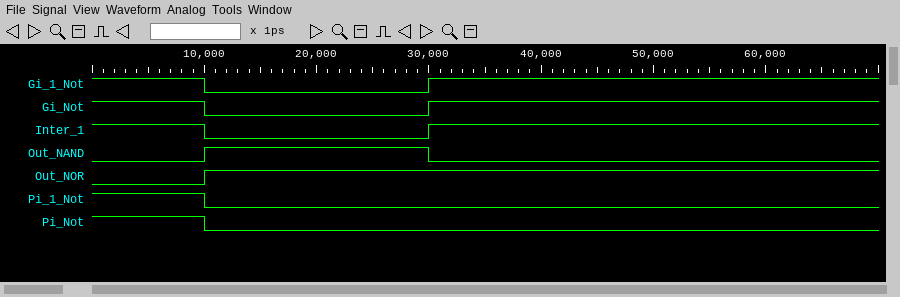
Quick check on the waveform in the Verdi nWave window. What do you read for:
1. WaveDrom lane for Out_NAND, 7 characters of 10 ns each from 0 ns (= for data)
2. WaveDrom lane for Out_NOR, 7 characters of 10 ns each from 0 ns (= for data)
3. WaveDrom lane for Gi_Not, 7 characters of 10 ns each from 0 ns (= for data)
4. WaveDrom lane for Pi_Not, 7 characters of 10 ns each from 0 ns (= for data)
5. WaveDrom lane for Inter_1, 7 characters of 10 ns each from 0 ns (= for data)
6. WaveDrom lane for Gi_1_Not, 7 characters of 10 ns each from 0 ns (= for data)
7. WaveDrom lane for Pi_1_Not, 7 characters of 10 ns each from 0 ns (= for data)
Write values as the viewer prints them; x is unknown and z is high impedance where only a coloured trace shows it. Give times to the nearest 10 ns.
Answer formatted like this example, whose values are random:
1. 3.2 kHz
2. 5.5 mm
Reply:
1. {name: 'Out_NAND', wave: '01.0...'}
2. {name: 'Out_NOR', wave: '01.....'}
3. {name: 'Gi_Not', wave: '10.1...'}
4. {name: 'Pi_Not', wave: '10.....'}
5. {name: 'Inter_1', wave: '10.1...'}
6. {name: 'Gi_1_Not', wave: '10.1...'}
7. {name: 'Pi_1_Not', wave: '10.....'}
